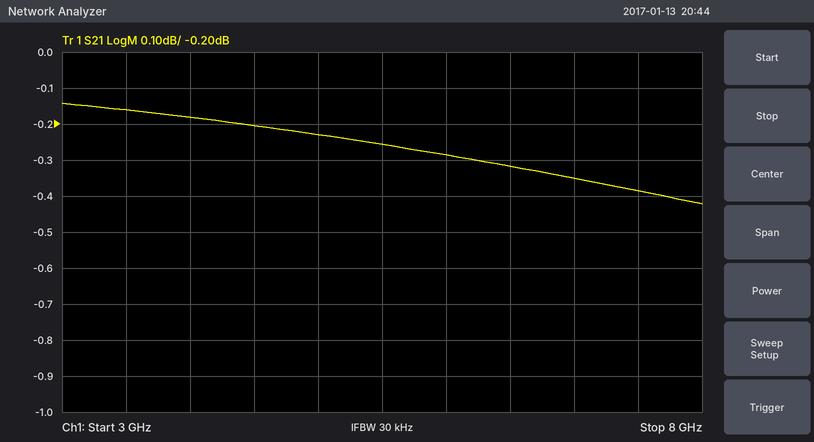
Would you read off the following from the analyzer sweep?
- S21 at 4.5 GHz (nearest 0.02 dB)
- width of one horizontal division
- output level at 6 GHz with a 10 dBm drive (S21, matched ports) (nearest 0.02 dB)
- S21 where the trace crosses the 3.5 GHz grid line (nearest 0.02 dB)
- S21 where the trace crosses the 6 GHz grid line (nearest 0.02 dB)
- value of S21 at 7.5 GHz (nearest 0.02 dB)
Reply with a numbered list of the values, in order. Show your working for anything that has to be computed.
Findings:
1. -0.20 dB
2. 500 MHz
3. 10 dBm + (-0.28 dB) = 9.72 dBm
4. -0.16 dB
5. -0.28 dB
6. -0.38 dB
